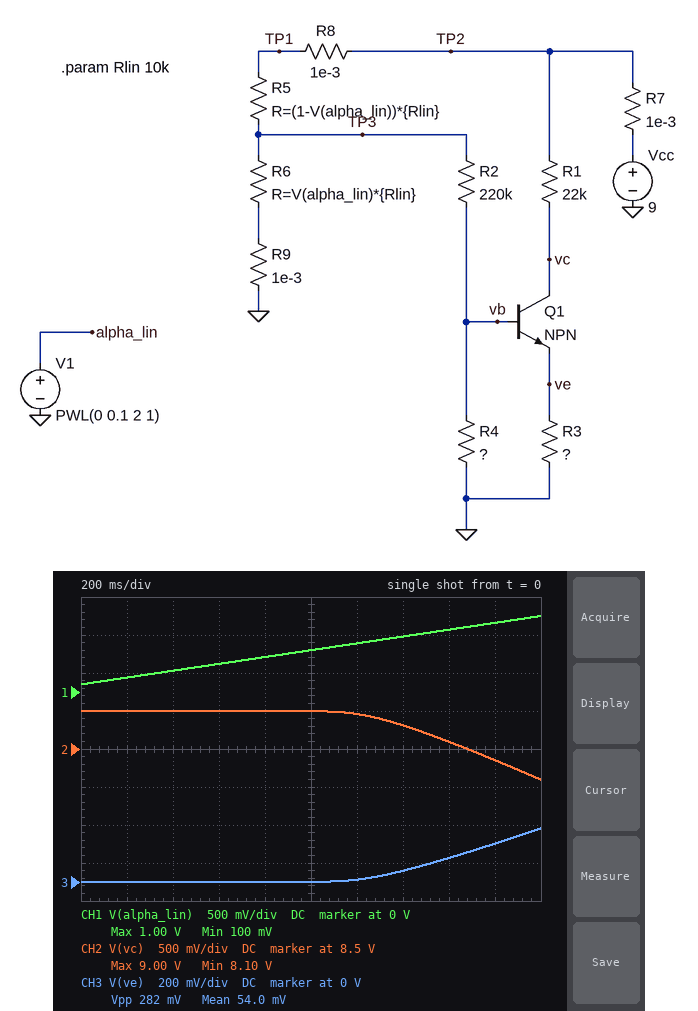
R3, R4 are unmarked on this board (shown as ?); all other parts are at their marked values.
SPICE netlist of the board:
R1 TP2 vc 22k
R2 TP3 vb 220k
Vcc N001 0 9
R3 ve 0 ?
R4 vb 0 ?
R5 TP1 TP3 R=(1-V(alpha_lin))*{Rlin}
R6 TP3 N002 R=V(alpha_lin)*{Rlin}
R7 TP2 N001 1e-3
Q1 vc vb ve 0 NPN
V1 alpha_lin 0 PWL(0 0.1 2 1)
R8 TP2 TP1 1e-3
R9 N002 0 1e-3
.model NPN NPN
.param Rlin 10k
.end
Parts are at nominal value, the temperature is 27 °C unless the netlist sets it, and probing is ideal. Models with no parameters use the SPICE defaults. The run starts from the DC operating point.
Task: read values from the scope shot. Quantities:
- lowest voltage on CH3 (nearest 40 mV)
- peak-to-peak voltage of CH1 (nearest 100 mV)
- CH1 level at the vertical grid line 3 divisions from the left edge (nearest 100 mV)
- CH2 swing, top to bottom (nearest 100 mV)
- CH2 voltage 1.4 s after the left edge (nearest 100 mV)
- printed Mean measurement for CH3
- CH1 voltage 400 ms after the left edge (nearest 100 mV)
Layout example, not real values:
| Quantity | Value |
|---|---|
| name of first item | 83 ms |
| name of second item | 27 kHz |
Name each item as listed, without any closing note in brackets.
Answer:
| Quantity | Value |
|---|---|
| lowest voltage on CH3 | 0 V |
| peak-to-peak voltage of CH1 | 900 mV |
| CH1 level at the vertical grid line 3 divisions from the left edge | 400 mV |
| CH2 swing, top to bottom | 900 mV |
| CH2 voltage 1.4 s after the left edge | 8.8 V |
| printed Mean measurement for CH3 | 54.0 mV |
| CH1 voltage 400 ms after the left edge | 300 mV |
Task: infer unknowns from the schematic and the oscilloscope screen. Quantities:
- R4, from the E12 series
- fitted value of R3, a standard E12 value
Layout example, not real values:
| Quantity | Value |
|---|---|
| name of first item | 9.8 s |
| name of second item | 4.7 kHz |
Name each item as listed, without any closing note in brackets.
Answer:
| Quantity | Value |
|---|---|
| R4, from the E12 series | 27 kΩ |
| fitted value of R3, a standard E12 value | 6.8 kΩ |
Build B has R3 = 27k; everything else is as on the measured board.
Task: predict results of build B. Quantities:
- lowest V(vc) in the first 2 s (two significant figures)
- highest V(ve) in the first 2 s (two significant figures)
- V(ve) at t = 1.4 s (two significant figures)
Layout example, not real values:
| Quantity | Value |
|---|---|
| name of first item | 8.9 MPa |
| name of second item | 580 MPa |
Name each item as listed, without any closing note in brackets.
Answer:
| Quantity | Value |
|---|---|
| lowest V(vc) in the first 2 s | 8.7 V |
| highest V(ve) in the first 2 s | 320 mV |
| V(ve) at t = 1.4 s | 86 mV |
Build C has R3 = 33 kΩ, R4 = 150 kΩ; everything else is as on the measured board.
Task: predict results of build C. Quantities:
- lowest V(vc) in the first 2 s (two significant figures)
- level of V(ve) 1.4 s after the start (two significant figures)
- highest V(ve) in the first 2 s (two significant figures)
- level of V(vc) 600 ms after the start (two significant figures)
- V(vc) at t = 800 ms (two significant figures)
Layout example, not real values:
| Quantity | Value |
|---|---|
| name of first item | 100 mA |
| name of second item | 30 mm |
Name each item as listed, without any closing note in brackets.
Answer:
| Quantity | Value |
|---|---|
| lowest V(vc) in the first 2 s | 7.1 V |
| level of V(ve) 1.4 s after the start | 1.9 V |
| highest V(ve) in the first 2 s | 2.9 V |
| level of V(vc) 600 ms after the start | 8.6 V |
| V(vc) at t = 800 ms | 8.4 V |
